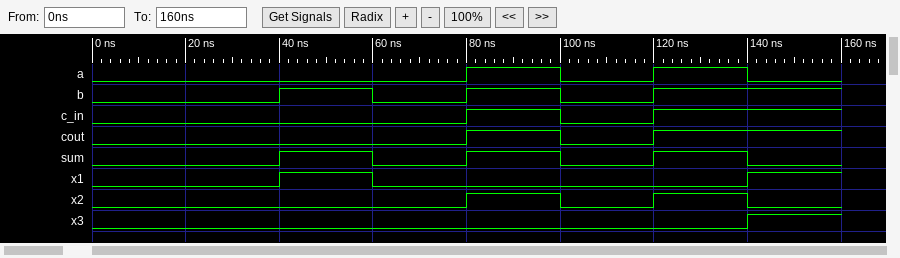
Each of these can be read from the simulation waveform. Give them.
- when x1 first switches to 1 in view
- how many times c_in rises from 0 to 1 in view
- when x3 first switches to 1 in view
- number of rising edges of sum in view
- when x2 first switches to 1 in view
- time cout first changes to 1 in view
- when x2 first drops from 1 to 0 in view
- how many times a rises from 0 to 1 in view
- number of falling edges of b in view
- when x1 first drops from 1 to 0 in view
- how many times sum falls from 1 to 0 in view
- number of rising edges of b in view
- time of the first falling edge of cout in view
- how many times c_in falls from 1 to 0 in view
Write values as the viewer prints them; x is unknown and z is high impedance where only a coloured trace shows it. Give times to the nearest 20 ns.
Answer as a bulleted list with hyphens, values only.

- 40 ns
- 2
- 140 ns
- 3
- 80 ns
- 80 ns
- 100 ns
- 2
- 2
- 60 ns
- 3
- 3
- 100 ns
- 1
